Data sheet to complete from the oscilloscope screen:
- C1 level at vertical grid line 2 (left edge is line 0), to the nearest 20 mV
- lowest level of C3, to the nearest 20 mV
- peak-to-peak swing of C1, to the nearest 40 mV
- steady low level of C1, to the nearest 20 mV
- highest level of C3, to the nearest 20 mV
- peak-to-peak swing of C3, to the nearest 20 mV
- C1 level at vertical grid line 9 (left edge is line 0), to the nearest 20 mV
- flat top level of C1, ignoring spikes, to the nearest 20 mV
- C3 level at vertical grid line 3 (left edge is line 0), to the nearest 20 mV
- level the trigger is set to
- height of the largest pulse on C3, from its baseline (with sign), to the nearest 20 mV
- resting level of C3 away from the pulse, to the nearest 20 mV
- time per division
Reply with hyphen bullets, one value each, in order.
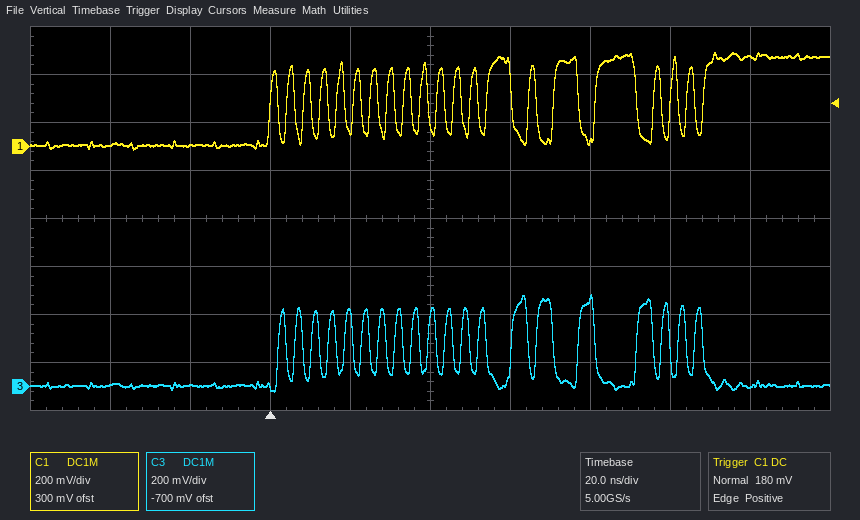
- 0 mV
- -20 mV
- 400 mV
- 0 mV
- 380 mV
- 400 mV
- 380 mV
- 380 mV
- 0 mV
- 180 mV
- +380 mV
- 0 mV
- 20 ns
